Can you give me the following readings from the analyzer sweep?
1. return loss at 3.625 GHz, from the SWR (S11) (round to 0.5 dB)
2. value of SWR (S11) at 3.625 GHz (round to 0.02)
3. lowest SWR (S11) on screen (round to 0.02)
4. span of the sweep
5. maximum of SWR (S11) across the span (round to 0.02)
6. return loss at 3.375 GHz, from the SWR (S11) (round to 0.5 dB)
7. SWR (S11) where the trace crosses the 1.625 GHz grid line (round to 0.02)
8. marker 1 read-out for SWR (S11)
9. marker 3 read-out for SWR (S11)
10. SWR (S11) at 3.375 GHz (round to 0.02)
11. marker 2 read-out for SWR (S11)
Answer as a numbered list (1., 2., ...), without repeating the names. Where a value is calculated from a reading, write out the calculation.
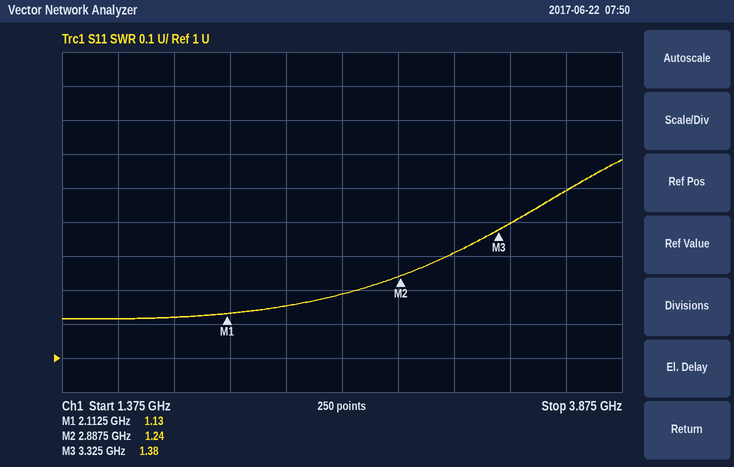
1. −20 log10((1.5 − 1)/(1.5 + 1)) ≈ 14.0 dB
2. 1.50
3. 1.12
4. 2.5 GHz
5. 1.58
6. −20 log10((1.4 − 1)/(1.4 + 1)) ≈ 15.6 dB, so 15.5 dB to the nearest 0.5 dB
7. 1.12
8. 1.13
9. 1.38
10. 1.40
11. 1.24
